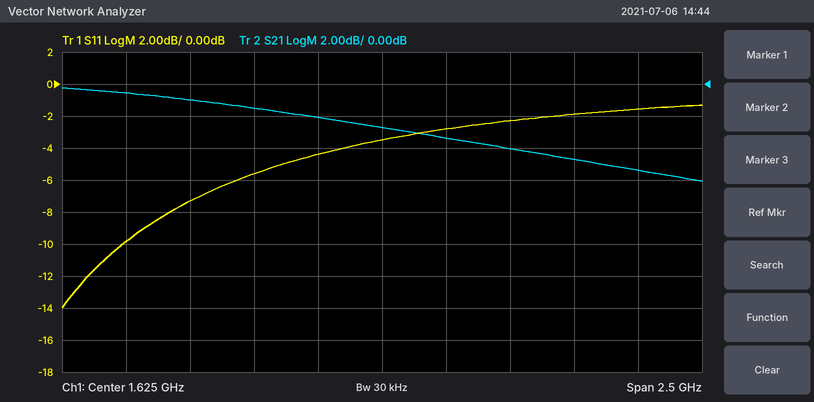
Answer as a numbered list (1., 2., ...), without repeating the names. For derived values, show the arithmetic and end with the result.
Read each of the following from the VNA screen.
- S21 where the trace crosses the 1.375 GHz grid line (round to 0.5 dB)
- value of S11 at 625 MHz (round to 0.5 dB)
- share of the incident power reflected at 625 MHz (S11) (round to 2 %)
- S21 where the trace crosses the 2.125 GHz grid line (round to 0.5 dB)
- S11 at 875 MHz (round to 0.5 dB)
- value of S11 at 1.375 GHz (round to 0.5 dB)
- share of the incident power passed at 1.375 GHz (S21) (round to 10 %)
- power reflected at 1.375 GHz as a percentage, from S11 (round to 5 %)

1. -2.0 dB
2. -10.0 dB
3. 10^(-10/10) ≈ 10 %
4. -4.0 dB
5. -7.5 dB
6. -4.5 dB
7. 10^(-2/10) ≈ 63.1 %, so 60 % to the nearest 10 %
8. 10^(-4.5/10) ≈ 35 %
